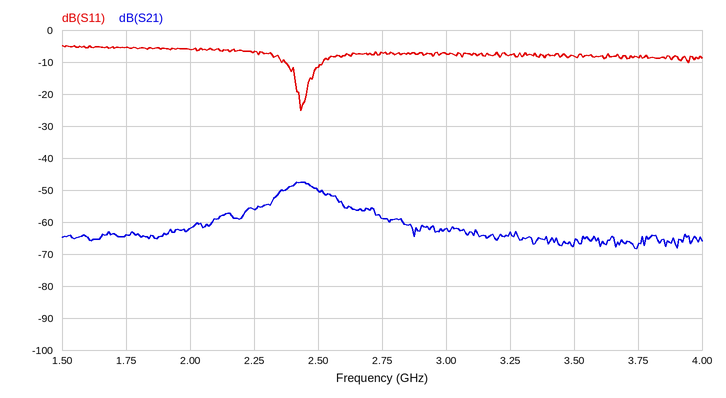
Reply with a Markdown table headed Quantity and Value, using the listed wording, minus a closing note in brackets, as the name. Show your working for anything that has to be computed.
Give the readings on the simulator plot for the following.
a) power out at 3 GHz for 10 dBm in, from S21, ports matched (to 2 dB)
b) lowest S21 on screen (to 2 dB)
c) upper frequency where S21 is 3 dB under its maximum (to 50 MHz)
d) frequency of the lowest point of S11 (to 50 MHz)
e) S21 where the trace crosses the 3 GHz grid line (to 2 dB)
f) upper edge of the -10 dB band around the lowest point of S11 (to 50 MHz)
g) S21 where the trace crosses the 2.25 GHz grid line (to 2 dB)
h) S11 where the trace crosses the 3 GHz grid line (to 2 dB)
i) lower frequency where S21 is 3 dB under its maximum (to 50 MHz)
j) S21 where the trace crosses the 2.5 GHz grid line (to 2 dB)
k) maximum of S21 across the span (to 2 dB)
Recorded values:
| Quantity | Value |
|---|---|
| power out at 3 GHz for 10 dBm in, from S21, ports matched | 10 dBm + (-62 dB) = -52 dBm |
| lowest S21 on screen | -68 dB |
| upper frequency where S21 is 3 dB under its maximum | 2.50 GHz |
| frequency of the lowest point of S11 | 2.45 GHz |
| S21 where the trace crosses the 3 GHz grid line | -62 dB |
| upper edge of the -10 dB band around the lowest point of S11 | 2.50 GHz |
| S21 where the trace crosses the 2.25 GHz grid line | -56 dB |
| S11 where the trace crosses the 3 GHz grid line | -8 dB |
| lower frequency where S21 is 3 dB under its maximum | 2.35 GHz |
| S21 where the trace crosses the 2.5 GHz grid line | -50 dB |
| maximum of S21 across the span | -48 dB |
